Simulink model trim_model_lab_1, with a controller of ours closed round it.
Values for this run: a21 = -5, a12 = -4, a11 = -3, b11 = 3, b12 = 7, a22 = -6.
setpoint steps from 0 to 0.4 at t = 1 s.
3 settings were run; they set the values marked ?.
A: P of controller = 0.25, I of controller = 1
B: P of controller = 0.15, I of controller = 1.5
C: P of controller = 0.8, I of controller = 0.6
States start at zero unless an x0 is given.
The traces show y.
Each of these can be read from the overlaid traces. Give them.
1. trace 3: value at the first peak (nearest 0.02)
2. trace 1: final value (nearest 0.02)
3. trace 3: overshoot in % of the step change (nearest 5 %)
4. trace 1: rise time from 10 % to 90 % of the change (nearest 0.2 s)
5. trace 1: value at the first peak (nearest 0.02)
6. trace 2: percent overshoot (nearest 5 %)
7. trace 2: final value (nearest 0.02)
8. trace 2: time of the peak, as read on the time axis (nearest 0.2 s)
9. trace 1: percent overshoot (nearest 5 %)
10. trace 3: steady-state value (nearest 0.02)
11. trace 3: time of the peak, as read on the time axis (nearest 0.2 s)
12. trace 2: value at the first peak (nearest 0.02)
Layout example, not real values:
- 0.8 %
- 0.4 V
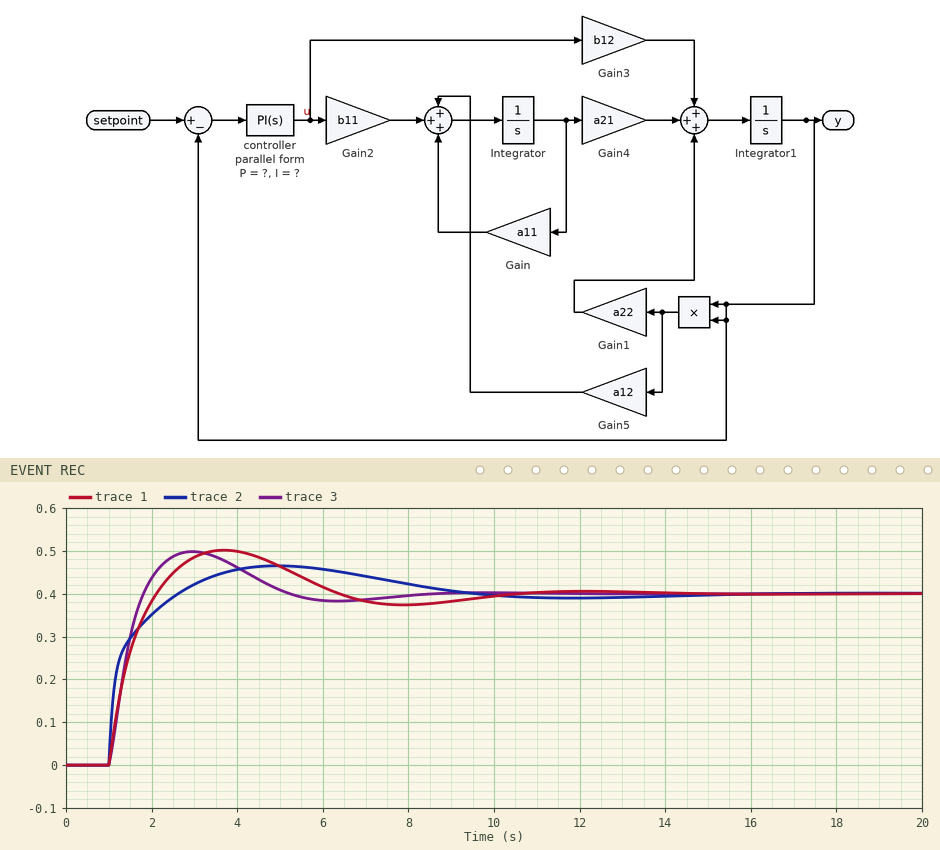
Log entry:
- 0.50
- 0.40
- 25 %
- 0.8 s
- 0.50
- 15 %
- 0.40
- 5.0 s
- 25 %
- 0.40
- 3.0 s
- 0.46
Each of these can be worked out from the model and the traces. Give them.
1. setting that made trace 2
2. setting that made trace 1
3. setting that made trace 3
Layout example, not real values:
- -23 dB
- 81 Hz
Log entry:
- C
- A
- B
